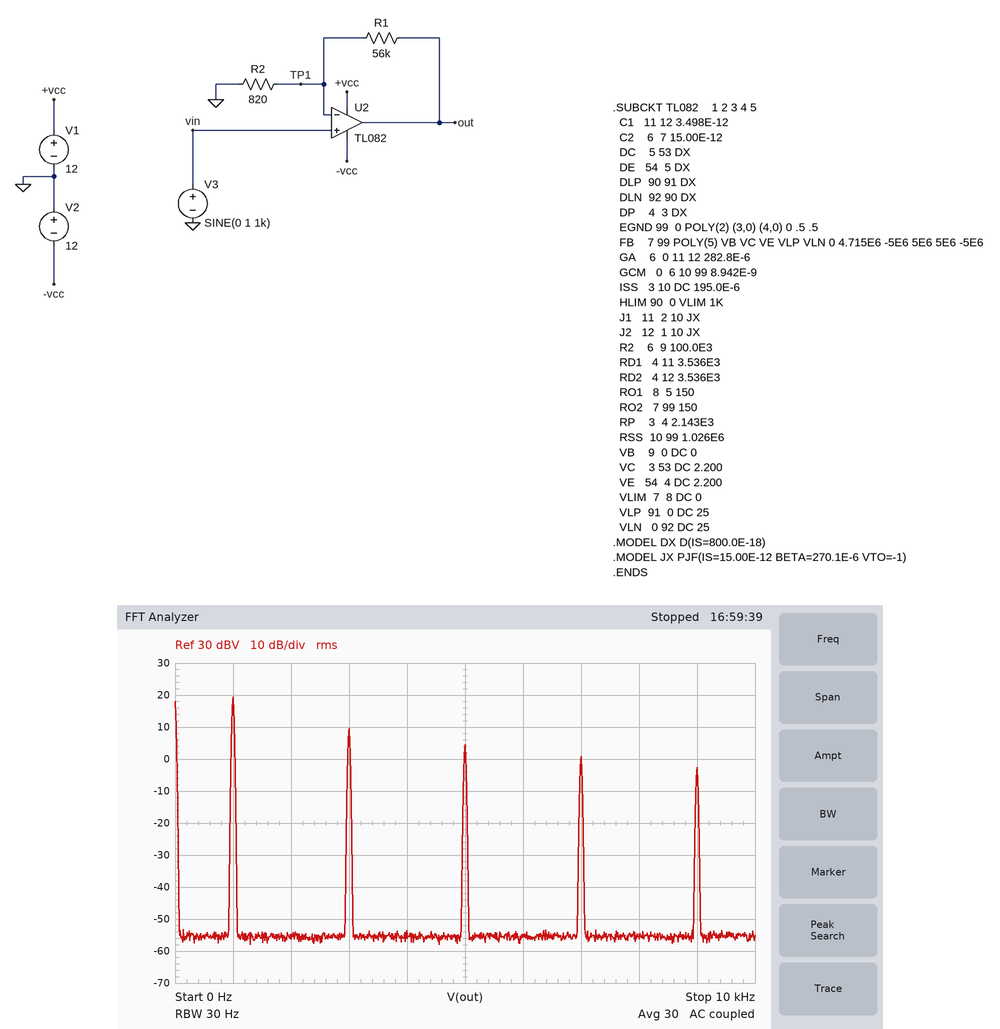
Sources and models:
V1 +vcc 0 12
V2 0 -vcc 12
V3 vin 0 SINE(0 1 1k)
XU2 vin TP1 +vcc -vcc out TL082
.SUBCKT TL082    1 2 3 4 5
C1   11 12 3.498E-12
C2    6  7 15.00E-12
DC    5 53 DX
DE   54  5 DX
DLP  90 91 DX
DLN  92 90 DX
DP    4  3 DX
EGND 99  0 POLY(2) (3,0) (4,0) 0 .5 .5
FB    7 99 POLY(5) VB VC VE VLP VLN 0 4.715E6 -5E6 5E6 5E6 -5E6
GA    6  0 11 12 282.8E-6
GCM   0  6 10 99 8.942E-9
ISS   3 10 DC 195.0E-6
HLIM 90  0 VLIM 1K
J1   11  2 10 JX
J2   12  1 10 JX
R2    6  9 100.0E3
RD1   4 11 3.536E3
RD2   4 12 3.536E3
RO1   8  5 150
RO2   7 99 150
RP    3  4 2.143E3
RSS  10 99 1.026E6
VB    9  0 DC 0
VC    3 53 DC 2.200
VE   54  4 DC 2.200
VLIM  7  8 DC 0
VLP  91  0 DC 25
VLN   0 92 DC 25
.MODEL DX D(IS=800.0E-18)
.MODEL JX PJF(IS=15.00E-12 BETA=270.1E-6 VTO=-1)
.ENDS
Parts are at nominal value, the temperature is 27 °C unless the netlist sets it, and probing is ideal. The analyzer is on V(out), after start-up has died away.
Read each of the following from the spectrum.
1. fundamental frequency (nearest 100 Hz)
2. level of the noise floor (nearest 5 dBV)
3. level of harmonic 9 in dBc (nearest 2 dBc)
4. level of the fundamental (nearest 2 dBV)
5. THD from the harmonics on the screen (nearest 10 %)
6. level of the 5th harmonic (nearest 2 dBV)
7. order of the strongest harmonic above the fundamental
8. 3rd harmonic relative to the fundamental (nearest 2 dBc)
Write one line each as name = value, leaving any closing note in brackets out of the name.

fundamental frequency = 1.0 kHz
level of the noise floor = -55 dBV
level of harmonic 9 in dBc = -22 dBc
level of the fundamental = 20 dBV
THD from the harmonics on the screen = 40 %
level of the 5th harmonic = 4 dBV
order of the strongest harmonic above the fundamental = 3
3rd harmonic relative to the fundamental = -10 dBc
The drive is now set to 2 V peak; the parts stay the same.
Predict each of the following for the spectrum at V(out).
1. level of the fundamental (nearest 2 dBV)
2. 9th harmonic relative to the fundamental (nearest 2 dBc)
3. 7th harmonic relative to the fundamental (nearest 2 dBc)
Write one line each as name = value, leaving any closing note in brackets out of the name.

level of the fundamental = 20 dBV
9th harmonic relative to the fundamental = -20 dBc
7th harmonic relative to the fundamental = -18 dBc
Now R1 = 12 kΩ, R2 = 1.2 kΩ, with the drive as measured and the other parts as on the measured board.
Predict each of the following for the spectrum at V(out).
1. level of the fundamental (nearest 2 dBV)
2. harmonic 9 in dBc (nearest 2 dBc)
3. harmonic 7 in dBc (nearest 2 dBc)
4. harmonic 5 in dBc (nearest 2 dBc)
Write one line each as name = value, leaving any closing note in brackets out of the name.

level of the fundamental = 18 dBV
harmonic 9 in dBc = -46 dBc
harmonic 7 in dBc = -42 dBc
harmonic 5 in dBc = -38 dBc
